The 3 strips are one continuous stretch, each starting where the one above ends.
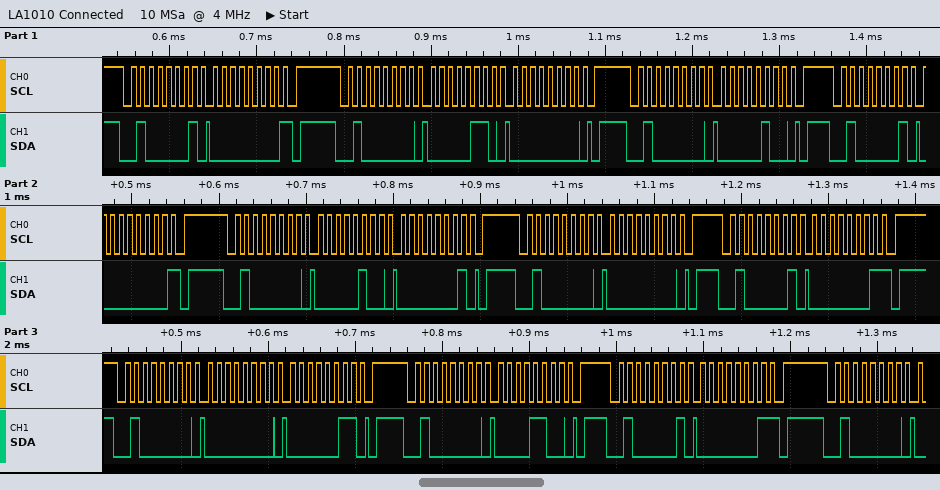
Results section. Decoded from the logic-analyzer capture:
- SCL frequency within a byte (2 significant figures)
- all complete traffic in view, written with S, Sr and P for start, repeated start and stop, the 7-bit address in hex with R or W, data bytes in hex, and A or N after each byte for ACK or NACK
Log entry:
100 kHz
S 20R A 00 N P S 20W A 06 A 00 A P S 20W A 04 A P S 20R A 00 N P S 20W A 04 A 01 A P S 20W A 00 A P S 20R A 01 N P S 20W A 00 A 03 A P S 20W A 0C A P S 20R A 01 N P S 20W A
